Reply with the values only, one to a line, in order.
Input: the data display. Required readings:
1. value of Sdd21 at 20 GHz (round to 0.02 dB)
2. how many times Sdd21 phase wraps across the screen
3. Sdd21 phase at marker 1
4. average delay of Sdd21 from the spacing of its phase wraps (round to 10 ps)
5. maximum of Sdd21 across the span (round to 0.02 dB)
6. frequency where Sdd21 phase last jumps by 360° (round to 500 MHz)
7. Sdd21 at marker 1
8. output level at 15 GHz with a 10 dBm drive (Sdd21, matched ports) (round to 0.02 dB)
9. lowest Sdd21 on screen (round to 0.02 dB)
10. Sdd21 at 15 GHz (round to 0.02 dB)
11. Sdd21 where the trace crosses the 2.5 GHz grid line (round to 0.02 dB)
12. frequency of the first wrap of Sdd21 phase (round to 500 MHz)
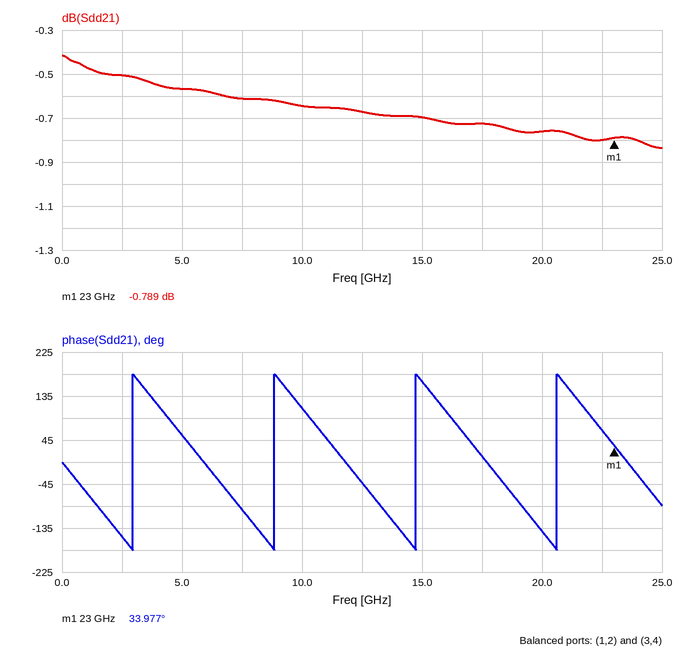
-0.76 dB
4
33.977°
170 ps
-0.42 dB
20.5 GHz
-0.789 dB
9.30 dBm
-0.84 dB
-0.70 dB
-0.50 dB
3.0 GHz
